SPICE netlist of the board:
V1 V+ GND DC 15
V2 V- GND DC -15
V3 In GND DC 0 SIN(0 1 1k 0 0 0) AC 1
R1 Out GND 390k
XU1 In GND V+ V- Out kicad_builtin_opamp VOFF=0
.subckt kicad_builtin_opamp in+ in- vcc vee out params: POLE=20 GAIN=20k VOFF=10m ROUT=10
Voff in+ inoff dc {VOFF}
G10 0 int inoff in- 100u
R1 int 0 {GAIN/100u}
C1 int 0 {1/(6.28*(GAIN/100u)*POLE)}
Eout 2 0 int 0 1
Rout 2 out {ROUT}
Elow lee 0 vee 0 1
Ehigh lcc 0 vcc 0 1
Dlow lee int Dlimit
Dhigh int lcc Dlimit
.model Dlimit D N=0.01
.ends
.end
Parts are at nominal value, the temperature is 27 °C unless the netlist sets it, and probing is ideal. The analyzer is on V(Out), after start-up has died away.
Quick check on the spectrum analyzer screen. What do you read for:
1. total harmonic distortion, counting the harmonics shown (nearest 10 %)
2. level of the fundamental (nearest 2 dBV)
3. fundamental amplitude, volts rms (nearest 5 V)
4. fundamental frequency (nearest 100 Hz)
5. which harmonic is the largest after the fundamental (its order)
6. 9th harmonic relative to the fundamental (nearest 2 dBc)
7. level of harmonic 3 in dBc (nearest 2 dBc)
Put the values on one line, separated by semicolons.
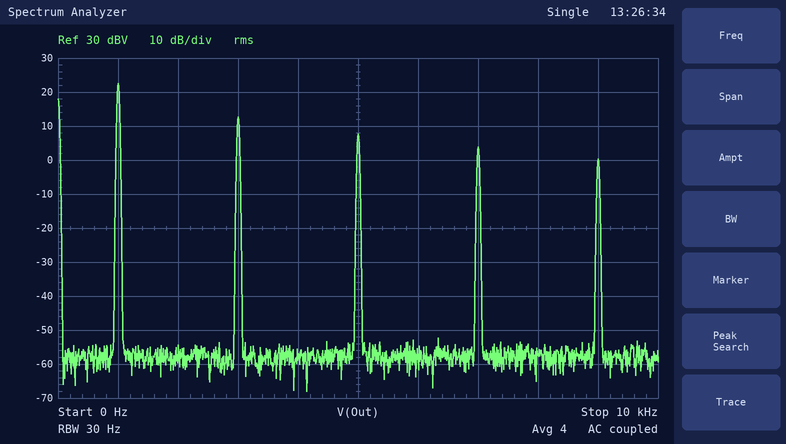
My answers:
40 %; 22 dBV; 15 V; 1.0 kHz; 3; -22 dBc; -10 dBc
